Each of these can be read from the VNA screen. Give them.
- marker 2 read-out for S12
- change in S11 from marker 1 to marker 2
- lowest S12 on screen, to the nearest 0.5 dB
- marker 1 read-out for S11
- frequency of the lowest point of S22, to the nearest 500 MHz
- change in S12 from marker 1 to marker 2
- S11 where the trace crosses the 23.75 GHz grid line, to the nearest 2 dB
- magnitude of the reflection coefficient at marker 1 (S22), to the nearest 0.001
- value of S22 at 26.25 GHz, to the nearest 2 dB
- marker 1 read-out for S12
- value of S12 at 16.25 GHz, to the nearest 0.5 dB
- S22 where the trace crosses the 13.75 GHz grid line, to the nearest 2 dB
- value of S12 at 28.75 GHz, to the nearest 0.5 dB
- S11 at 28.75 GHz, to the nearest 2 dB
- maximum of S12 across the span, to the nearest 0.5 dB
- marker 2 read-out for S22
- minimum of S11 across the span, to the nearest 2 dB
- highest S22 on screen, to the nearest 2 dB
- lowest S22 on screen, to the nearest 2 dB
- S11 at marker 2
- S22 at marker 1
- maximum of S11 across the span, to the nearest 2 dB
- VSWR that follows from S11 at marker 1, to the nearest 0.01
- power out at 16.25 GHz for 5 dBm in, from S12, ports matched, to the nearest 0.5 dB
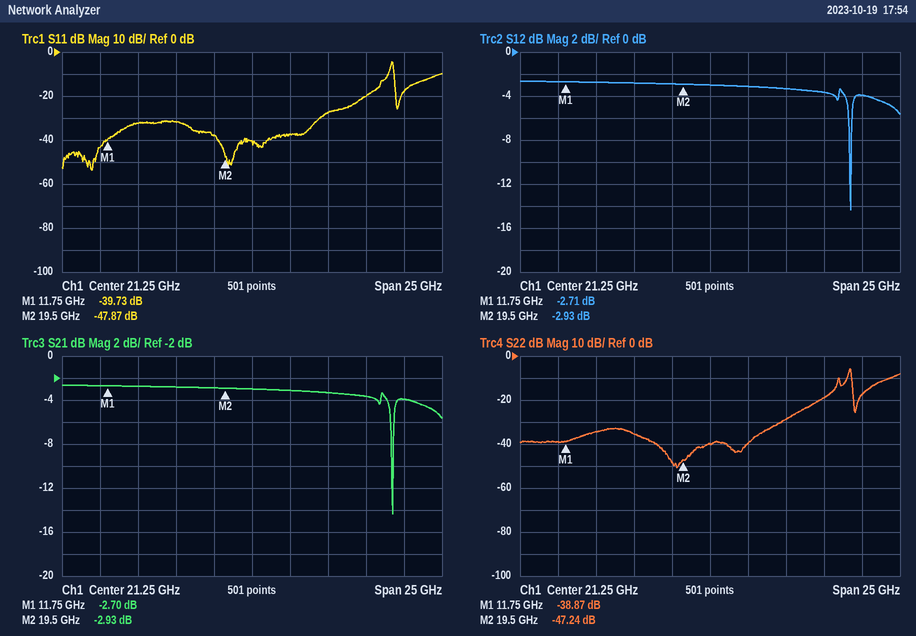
-2.93 dB
-8.14 dB
-14.5 dB
-39.73 dB
19.0 GHz
-0.22 dB
-38 dB
0.011
-28 dB
-2.71 dB
-3.0 dB
-34 dB
-3.5 dB
-20 dB
-2.5 dB
-47.24 dB
-54 dB
-6 dB
-50 dB
-47.87 dB
-38.87 dB
-4 dB
1.02
2.0 dBm
